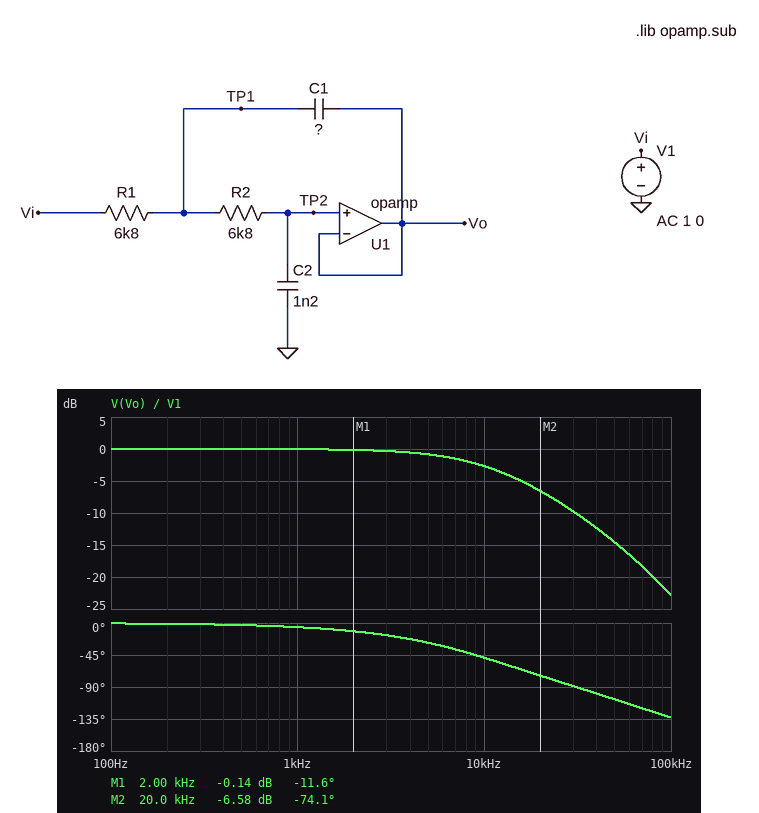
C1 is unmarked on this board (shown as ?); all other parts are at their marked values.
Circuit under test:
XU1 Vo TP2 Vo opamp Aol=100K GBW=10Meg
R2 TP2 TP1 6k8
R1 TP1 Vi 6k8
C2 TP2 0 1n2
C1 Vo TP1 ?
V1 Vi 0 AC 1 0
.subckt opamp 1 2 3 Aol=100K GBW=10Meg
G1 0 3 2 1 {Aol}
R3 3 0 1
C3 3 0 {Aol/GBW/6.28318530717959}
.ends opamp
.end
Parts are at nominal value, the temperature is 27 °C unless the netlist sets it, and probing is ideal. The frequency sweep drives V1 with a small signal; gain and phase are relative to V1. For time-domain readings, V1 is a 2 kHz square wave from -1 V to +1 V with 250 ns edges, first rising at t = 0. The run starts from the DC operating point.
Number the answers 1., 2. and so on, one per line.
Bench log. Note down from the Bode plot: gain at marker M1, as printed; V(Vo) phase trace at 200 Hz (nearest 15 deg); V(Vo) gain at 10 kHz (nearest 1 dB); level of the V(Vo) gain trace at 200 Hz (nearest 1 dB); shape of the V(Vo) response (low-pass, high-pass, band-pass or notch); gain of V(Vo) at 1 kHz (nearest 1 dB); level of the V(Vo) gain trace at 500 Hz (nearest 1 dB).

1. -0.14 dB
2. 0 deg
3. -3 dB
4. 0 dB
5. low-pass
6. 0 dB
7. 0 dB
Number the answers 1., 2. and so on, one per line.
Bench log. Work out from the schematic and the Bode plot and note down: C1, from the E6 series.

1. 470 pF
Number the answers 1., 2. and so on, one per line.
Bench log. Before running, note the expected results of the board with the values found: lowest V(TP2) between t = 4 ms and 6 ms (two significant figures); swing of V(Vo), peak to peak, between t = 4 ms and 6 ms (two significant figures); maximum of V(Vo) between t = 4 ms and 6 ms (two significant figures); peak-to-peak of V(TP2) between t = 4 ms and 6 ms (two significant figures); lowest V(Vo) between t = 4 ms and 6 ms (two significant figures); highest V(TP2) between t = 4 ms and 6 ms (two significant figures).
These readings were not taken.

1. -1.0 V
2. 2.0 V
3. 1.0 V
4. 2.0 V
5. -1.0 V
6. 1.0 V
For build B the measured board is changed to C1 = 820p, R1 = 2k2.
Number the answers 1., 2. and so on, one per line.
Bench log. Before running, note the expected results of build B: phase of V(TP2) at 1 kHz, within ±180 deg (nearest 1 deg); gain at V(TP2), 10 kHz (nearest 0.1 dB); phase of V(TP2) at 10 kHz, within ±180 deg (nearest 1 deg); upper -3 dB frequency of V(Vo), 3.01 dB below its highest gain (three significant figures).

1. -4 deg
2. -1.3 dB
3. -36 deg
4. 16.8 kHz
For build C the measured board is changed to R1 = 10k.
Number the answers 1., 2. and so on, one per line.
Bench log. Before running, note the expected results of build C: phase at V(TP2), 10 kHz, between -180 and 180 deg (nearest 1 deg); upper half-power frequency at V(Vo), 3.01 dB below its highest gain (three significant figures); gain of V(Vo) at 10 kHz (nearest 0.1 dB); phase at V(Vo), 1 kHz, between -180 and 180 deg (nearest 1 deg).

1. -56 deg
2. 8.71 kHz
3. -3.7 dB
4. -7 deg
